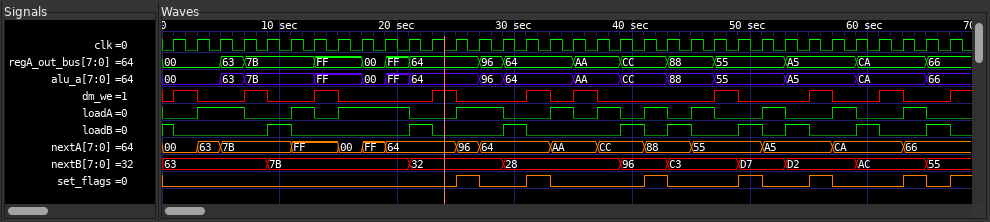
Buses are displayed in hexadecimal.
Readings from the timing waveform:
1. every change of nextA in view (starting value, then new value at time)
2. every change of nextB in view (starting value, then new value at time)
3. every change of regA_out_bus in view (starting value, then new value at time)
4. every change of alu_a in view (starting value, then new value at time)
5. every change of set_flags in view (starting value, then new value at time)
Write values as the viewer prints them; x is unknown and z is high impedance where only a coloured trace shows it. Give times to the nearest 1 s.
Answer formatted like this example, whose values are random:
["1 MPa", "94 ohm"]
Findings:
["00, 63 at 3 s, 7B at 5 s, FF at 11 s, 00 at 15 s, FF at 17 s, 64 at 19 s, 96 at 25 s, 64 at 27 s, AA at 33 s, CC at 37 s, 88 at 41 s, 55 at 45 s, A5 at 51 s, CA at 57 s, 66 at 63 s", "63, 7B at 9 s, 32 at 21 s, 28 at 29 s, 96 at 39 s, C3 at 43 s, D7 at 49 s, D2 at 53 s, AC at 59 s, 55 at 65 s", "00, 63 at 5 s, 7B at 7 s, FF at 13 s, 00 at 17 s, FF at 19 s, 64 at 21 s, 96 at 27 s, 64 at 29 s, AA at 35 s, CC at 39 s, 88 at 43 s, 55 at 47 s, A5 at 53 s, CA at 59 s, 66 at 65 s", "00, 63 at 5 s, 7B at 7 s, FF at 13 s, 00 at 17 s, FF at 19 s, 64 at 21 s, 96 at 27 s, 64 at 29 s, AA at 35 s, CC at 39 s, 88 at 43 s, 55 at 47 s, A5 at 53 s, CA at 59 s, 66 at 65 s", "0, 1 at 25 s, 0 at 27 s, 1 at 31 s, 0 at 33 s, 1 at 41 s, 0 at 43 s, 1 at 49 s, 0 at 51 s, 1 at 55 s, 0 at 57 s, 1 at 63 s, 0 at 65 s, 1 at 67 s"]
